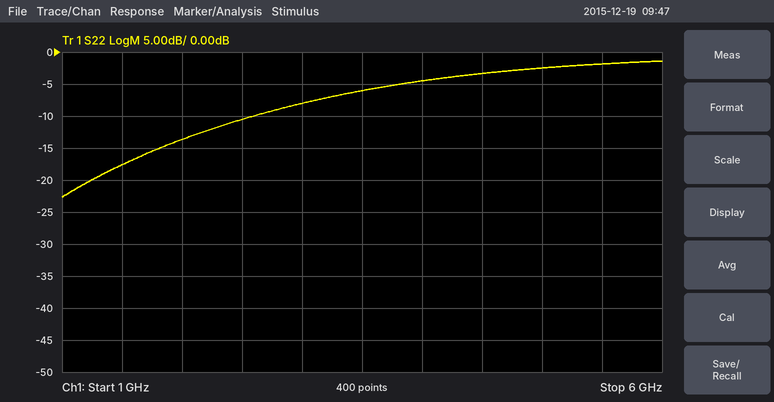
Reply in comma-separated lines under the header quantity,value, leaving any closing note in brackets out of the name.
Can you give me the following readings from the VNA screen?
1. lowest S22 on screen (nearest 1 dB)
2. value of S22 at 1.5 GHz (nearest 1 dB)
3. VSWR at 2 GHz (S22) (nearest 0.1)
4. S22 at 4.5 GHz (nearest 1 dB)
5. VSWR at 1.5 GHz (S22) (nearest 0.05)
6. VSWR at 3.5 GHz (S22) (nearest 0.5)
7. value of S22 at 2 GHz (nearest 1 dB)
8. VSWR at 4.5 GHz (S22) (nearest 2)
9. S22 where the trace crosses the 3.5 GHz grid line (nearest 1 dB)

quantity,value
lowest S22 on screen,-23 dB
value of S22 at 1.5 GHz,-18 dB
VSWR at 2 GHz (S22),1.5
S22 at 4.5 GHz,-3 dB
VSWR at 1.5 GHz (S22),1.30
VSWR at 3.5 GHz (S22),3.0
value of S22 at 2 GHz,-14 dB
VSWR at 4.5 GHz (S22),6
S22 where the trace crosses the 3.5 GHz grid line,-6 dB
